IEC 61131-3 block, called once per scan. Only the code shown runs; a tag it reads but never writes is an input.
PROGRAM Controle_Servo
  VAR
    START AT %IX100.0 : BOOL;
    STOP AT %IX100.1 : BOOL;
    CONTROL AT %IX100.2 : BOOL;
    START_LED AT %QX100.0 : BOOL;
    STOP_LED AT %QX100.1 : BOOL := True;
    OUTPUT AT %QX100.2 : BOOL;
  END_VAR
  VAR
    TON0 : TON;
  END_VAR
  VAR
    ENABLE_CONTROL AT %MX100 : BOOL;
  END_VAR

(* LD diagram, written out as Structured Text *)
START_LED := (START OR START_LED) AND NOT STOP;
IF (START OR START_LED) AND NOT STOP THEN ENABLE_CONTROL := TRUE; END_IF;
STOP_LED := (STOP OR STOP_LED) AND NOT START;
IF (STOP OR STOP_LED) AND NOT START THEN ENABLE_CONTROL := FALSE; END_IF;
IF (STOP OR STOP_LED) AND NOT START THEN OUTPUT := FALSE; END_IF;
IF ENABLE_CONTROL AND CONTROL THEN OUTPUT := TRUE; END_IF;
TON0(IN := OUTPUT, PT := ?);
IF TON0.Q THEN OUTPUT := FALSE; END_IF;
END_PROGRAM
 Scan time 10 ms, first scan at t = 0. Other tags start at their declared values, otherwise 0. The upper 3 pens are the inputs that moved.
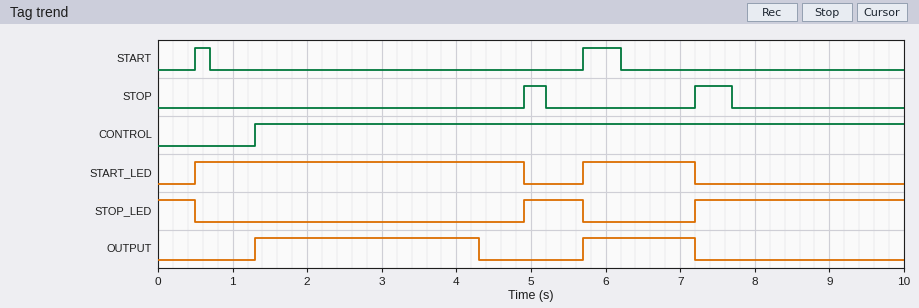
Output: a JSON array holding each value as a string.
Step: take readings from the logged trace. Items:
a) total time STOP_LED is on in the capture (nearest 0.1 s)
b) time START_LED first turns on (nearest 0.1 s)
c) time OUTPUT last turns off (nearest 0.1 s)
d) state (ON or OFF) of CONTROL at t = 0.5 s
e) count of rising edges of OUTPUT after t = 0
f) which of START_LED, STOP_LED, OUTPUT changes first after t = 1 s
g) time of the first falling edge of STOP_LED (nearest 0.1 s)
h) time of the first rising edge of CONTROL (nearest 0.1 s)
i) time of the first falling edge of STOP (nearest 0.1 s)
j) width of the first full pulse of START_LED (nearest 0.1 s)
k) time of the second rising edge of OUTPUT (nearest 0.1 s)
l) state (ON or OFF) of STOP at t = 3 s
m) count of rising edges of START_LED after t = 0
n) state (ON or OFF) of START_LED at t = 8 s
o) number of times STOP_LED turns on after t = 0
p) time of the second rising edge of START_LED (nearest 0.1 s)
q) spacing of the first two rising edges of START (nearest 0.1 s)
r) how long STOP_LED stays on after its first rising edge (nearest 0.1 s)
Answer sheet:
["4.1 s", "0.5 s", "7.2 s", "OFF", "2", "OUTPUT", "0.5 s", "1.3 s", "5.2 s", "4.4 s", "5.7 s", "OFF", "2", "OFF", "2", "5.7 s", "5.2 s", "0.8 s"]
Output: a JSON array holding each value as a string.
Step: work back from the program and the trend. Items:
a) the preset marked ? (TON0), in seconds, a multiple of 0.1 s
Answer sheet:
["3.0 s"]
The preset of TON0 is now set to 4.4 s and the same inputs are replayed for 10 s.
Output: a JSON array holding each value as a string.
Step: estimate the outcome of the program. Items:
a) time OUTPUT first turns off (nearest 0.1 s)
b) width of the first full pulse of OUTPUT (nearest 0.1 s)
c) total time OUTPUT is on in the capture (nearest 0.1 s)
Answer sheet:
["4.9 s", "3.6 s", "5.1 s"]
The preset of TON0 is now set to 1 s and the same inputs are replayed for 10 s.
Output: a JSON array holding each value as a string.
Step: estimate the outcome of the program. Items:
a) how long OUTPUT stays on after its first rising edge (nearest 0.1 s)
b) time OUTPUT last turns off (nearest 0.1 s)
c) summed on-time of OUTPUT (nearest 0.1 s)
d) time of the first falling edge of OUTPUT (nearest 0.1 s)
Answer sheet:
["1.0 s", "6.7 s", "2.0 s", "2.3 s"]
